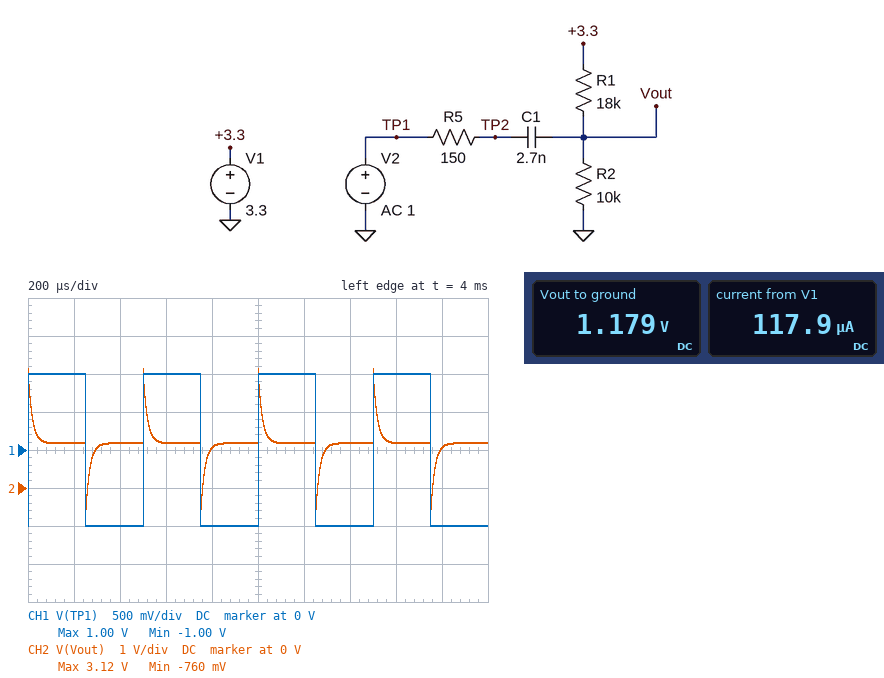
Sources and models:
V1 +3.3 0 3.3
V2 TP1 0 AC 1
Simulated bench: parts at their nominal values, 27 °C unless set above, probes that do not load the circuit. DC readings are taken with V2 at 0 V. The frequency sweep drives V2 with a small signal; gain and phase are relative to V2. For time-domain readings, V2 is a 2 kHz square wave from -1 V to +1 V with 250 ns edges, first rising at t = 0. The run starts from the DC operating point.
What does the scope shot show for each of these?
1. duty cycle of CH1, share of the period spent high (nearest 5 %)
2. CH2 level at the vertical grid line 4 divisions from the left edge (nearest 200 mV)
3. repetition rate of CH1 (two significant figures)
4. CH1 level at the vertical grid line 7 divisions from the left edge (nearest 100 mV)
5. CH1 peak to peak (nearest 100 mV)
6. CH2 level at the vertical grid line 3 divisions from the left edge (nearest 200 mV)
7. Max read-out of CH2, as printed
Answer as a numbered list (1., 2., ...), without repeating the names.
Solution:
1. 50 %
2. 1.0 V
3. 2.0 kHz
4. -1.0 V
5. 2.0 V
6. 1.2 V
7. 3.12 V
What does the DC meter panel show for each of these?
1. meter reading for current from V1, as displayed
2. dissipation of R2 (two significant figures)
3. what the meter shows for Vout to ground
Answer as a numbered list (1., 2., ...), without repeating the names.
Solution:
1. 117.9 µA
2. 140 µW
3. 1.179 V
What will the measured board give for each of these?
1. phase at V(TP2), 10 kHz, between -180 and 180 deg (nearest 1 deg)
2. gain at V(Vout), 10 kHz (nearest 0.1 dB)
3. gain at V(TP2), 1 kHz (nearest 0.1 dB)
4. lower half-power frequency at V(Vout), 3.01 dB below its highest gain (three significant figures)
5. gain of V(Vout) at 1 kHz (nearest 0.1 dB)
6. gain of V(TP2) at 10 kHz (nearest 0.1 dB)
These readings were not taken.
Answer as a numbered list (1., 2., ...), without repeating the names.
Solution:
1. -1 deg
2. -2.8 dB
3. 0 dB
4. 8.96 kHz
5. -19.3 dB
6. -0.1 dB
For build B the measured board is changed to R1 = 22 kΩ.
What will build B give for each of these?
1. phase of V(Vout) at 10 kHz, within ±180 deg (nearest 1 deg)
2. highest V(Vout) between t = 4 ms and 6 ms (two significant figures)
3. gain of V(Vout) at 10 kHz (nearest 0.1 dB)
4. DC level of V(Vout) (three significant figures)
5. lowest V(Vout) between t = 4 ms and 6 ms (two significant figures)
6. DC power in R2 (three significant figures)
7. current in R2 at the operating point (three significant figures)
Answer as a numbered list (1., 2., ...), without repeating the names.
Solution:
1. 40 deg
2. 3.0 V
3. -2.5 dB
4. 1.03 V
5. -910 mV
6. 106 µW
7. 103 µA
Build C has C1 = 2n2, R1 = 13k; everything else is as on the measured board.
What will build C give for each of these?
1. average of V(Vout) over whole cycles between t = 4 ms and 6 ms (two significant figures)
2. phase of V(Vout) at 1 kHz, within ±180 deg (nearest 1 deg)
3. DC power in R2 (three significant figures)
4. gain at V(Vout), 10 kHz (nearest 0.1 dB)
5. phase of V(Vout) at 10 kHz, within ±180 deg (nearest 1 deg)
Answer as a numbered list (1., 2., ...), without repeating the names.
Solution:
1. 1.4 V
2. 85 deg
3. 206 µW
4. -4.3 dB
5. 51 deg
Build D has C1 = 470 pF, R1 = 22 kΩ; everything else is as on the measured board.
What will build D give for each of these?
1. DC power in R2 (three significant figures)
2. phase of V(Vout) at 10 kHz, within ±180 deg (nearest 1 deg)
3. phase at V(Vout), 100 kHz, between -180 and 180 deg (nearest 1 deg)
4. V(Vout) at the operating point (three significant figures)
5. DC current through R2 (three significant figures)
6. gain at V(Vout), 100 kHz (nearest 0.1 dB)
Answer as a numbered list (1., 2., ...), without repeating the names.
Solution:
1. 106 µW
2. 78 deg
3. 26 deg
4. 1.03 V
5. 103 µA
6. -1.1 dB
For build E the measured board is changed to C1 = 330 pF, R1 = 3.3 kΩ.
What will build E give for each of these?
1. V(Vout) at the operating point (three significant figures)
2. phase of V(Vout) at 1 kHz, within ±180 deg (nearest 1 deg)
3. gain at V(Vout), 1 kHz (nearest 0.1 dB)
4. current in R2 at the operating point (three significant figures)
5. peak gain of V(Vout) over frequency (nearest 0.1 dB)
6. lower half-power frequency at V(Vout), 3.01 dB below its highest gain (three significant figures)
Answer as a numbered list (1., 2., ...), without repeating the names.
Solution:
1. 2.48 V
2. 90 deg
3. -45.8 dB
4. 248 µA
5. -0.5 dB
6. 183 kHz
